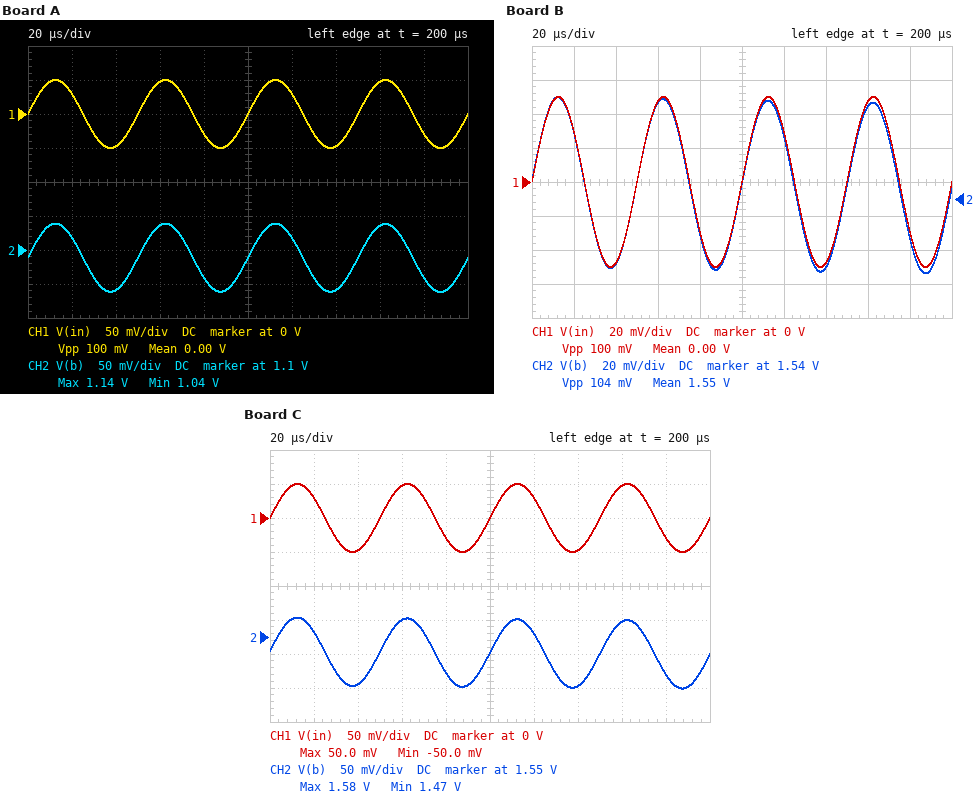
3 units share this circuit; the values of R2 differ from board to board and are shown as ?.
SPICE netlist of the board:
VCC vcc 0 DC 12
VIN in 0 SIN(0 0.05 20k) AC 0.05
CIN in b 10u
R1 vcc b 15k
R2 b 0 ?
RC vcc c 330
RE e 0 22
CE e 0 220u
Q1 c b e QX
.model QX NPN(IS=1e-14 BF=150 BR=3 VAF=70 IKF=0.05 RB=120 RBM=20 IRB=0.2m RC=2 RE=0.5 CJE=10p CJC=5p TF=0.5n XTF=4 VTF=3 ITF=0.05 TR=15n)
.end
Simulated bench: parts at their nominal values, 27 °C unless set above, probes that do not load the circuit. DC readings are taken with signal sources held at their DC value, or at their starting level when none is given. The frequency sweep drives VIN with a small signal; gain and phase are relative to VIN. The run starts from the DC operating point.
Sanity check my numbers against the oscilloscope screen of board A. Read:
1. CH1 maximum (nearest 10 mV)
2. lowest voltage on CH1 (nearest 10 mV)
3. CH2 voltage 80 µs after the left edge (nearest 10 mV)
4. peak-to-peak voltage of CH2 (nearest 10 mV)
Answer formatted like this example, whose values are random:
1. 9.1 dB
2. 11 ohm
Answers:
1. 50 mV
2. -50 mV
3. 1.06 V
4. 100 mV
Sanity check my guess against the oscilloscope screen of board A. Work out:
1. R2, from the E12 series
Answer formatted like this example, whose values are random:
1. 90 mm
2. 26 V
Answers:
1. 1.8 kΩ
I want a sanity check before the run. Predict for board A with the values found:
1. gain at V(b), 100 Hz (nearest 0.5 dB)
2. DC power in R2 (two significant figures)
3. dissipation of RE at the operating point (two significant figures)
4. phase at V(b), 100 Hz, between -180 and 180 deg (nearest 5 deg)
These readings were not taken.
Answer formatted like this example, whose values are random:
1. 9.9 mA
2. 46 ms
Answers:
1. -1.5 dB
2. 660 µW
3. 5.3 mW
4. 10 deg
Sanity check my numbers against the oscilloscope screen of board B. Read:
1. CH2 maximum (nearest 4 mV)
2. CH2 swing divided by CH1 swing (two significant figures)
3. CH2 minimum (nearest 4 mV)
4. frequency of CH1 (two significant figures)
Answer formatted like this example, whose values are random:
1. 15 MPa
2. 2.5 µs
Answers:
1. 1.600 V
2. 1.0
3. 1.496 V
4. 20 kHz
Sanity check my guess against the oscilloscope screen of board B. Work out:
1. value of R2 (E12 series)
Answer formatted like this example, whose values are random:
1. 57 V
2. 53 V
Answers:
1. 10 kΩ
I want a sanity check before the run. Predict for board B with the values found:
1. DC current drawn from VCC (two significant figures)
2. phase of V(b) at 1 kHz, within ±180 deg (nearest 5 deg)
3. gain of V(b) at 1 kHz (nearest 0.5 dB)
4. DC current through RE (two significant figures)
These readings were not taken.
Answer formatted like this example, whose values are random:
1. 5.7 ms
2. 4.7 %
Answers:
1. 34 mA
2. 15 deg
3. -0.5 dB
4. 34 mA
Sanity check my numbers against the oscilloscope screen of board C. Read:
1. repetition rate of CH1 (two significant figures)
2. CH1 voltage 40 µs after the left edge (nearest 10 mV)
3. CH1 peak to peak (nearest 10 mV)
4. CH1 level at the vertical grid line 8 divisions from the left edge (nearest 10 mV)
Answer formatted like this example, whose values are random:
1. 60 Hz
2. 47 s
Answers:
1. 20 kHz
2. -50 mV
3. 100 mV
4. 50 mV
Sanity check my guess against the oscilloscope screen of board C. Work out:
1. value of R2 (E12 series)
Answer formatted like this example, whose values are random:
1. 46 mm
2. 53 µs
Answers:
1. 4.7 kΩ
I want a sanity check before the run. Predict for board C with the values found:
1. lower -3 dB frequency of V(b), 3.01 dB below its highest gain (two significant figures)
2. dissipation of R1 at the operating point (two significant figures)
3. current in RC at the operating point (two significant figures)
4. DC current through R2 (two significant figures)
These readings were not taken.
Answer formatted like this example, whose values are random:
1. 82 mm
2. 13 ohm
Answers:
1. 120 Hz
2. 7.3 mW
3. 33 mA
4. 330 µA
